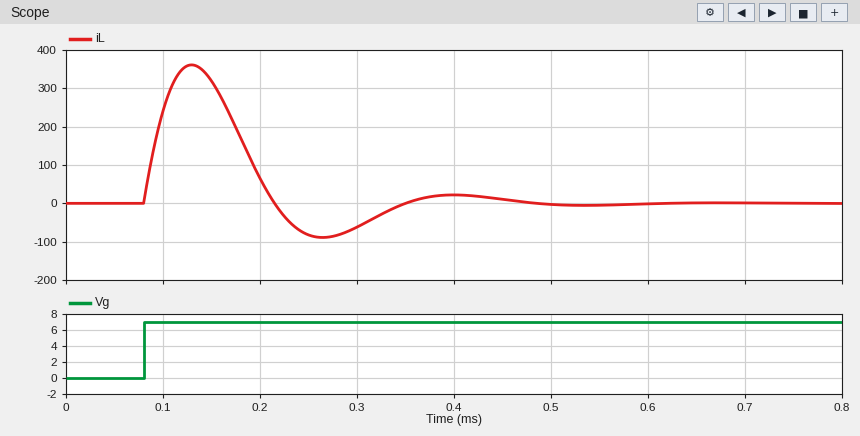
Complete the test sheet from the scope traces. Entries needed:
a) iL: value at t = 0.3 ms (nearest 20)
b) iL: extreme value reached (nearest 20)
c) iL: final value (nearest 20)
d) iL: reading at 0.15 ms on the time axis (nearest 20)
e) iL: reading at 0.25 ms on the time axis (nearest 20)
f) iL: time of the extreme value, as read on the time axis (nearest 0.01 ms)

-60
360
0
320
-80
0.13 ms
